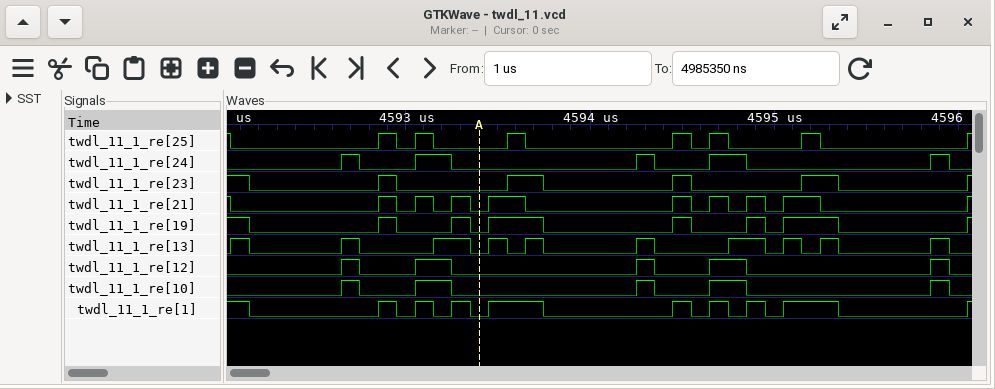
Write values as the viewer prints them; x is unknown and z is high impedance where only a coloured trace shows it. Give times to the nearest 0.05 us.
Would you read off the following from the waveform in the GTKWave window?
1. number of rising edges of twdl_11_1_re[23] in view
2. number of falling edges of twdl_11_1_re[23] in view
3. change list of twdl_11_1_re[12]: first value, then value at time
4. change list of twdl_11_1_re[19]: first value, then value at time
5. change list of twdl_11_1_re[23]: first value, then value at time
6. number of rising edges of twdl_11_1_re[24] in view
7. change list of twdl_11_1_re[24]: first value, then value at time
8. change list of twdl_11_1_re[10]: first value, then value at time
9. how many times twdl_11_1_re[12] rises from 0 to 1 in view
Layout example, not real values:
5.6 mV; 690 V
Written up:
5; 5; 0, 1 at 4592.65 us, 0 at 4592.75 us, 1 at 4593.05 us, 0 at 4593.25 us, 1 at 4594.25 us, 0 at 4594.35 us, 1 at 4594.65 us, 0 at 4594.85 us, 1 at 4595.85 us, 0 at 4595.95 us; 1, 0 at 4592.15 us, 1 at 4592.85 us, 0 at 4592.95 us, 1 at 4593.25 us, 0 at 4593.35 us, 1 at 4593.45 us, 0 at 4593.75 us, 1 at 4594.45 us, 0 at 4594.55 us, 1 at 4594.85 us, 0 at 4594.95 us, 1 at 4595.05 us, 0 at 4595.35 us, 1 at 4596.05 us; 1, 0 at 4592.15 us, 1 at 4592.85 us, 0 at 4592.95 us, 1 at 4593.55 us, 0 at 4593.75 us, 1 at 4594.45 us, 0 at 4594.55 us, 1 at 4595.15 us, 0 at 4595.35 us, 1 at 4596.05 us; 5; 0, 1 at 4592.65 us, 0 at 4592.75 us, 1 at 4593.05 us, 0 at 4593.25 us, 1 at 4594.25 us, 0 at 4594.35 us, 1 at 4594.65 us, 0 at 4594.85 us, 1 at 4595.85 us, 0 at 4595.95 us; 0, 1 at 4592.65 us, 0 at 4592.75 us, 1 at 4593.05 us, 0 at 4593.25 us, 1 at 4594.25 us, 0 at 4594.35 us, 1 at 4594.65 us, 0 at 4594.85 us, 1 at 4595.85 us, 0 at 4595.95 us; 5
